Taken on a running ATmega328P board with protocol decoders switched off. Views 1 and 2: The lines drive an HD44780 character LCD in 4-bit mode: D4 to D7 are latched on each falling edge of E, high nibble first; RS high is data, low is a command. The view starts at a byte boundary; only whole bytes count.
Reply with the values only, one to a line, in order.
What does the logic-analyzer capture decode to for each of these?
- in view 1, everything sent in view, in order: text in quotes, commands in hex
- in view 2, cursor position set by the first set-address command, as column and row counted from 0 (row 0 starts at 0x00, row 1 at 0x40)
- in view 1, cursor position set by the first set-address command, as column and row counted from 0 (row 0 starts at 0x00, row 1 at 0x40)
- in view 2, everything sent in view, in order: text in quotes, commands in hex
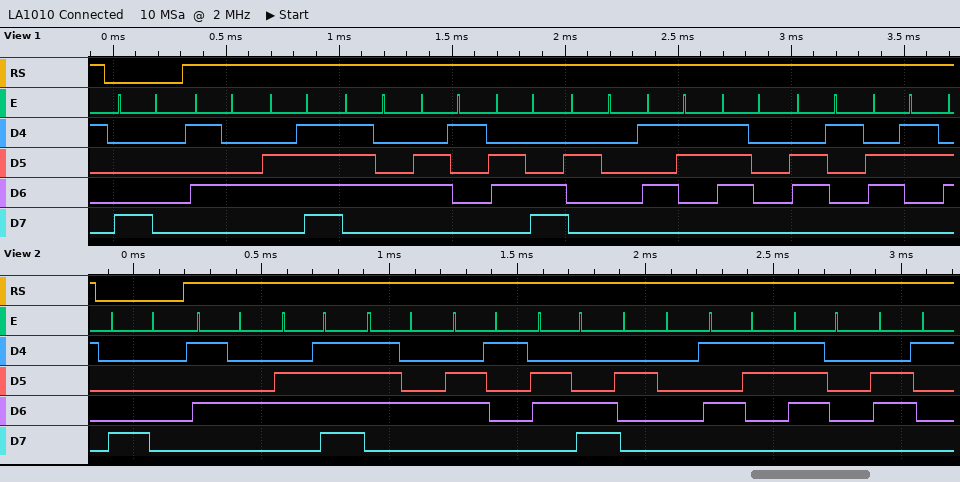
0x80 "Total Spac"
column 0, row 0
column 0, row 0
0x80 "Total Spa"
